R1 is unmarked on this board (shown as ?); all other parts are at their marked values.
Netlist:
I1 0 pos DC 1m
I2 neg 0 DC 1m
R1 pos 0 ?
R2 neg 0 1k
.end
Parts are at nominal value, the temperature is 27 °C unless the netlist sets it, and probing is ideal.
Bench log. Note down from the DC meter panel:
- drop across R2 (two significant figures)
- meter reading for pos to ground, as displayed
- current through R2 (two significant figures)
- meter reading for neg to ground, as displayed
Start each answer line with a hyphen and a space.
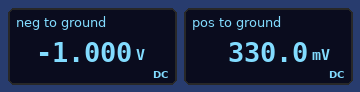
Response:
- 1.0 V
- 330.0 mV
- 1.0 mA
- -1.000 V
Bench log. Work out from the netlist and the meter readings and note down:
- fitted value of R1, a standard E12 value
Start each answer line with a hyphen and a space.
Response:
- 330 Ω
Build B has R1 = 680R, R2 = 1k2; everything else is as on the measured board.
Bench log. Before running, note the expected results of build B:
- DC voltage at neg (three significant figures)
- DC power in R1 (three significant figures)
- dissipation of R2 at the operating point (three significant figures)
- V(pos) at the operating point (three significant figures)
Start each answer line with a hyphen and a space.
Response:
- -1.20 V
- 680 µW
- 1.20 mW
- 680 mV
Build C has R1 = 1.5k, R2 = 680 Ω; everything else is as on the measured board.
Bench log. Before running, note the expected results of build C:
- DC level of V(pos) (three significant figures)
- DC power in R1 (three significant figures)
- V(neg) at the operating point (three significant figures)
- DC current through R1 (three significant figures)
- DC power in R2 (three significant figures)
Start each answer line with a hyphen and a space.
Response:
- 1.50 V
- 1.50 mW
- -680 mV
- 1.00 mA
- 680 µW
